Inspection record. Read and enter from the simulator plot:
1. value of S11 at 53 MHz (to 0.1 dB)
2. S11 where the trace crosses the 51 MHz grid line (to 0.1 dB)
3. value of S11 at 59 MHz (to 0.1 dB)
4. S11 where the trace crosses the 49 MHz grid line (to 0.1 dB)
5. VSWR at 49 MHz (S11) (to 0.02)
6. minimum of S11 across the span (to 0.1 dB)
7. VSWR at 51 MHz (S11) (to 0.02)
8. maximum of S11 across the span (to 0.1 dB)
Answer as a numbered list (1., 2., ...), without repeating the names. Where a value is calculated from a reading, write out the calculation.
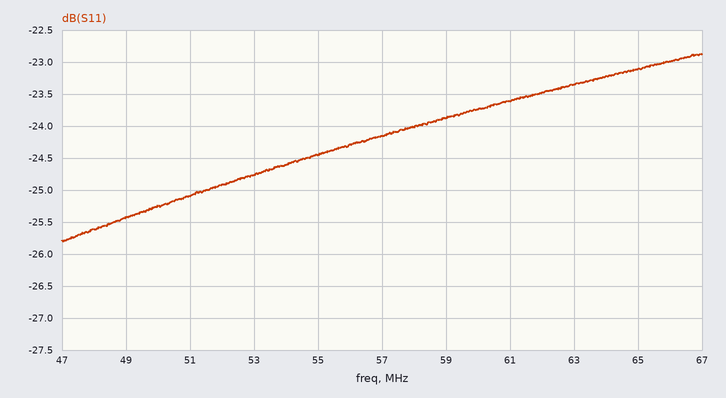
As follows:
1. -24.8 dB
2. -25.1 dB
3. -23.9 dB
4. -25.4 dB
5. |Γ| = 10^(-25.4/20) = 0.0537; VSWR = (1 + 0.0537)/(1 − 0.0537) ≈ 1.11, so 1.12 to the nearest 0.02
6. -25.8 dB
7. |Γ| = 10^(-25.1/20) = 0.0556; VSWR = (1 + 0.0556)/(1 − 0.0556) ≈ 1.12
8. -22.9 dB
